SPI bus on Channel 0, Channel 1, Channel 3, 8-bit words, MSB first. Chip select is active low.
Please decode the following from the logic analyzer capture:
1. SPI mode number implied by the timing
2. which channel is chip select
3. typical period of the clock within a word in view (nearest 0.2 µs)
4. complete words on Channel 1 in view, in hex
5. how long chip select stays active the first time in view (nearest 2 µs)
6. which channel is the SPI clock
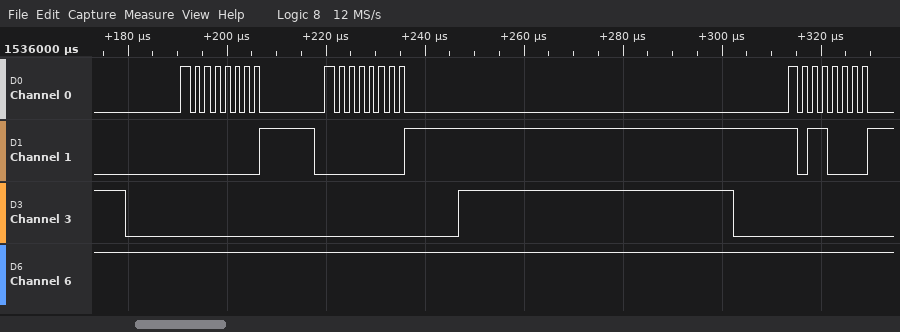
0
Channel 3
2 µs
00, 00, B0
68 µs
Channel 0
